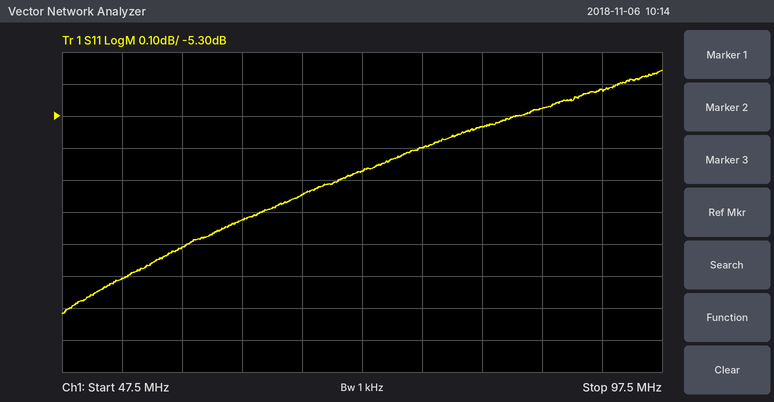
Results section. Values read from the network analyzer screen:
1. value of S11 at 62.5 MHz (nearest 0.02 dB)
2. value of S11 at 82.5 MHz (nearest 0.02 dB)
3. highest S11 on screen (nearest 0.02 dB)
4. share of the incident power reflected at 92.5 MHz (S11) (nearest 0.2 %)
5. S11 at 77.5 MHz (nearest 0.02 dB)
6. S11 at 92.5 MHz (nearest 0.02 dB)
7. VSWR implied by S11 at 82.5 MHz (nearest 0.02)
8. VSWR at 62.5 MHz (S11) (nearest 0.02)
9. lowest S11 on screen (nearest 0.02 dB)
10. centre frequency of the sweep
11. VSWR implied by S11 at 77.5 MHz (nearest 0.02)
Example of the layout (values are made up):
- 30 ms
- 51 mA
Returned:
- -5.62 dB
- -5.34 dB
- -5.16 dB
- 30.0 %
- -5.40 dB
- -5.22 dB
- 3.36
- 3.20
- -5.92 dB
- 72.5 MHz
- 3.32
